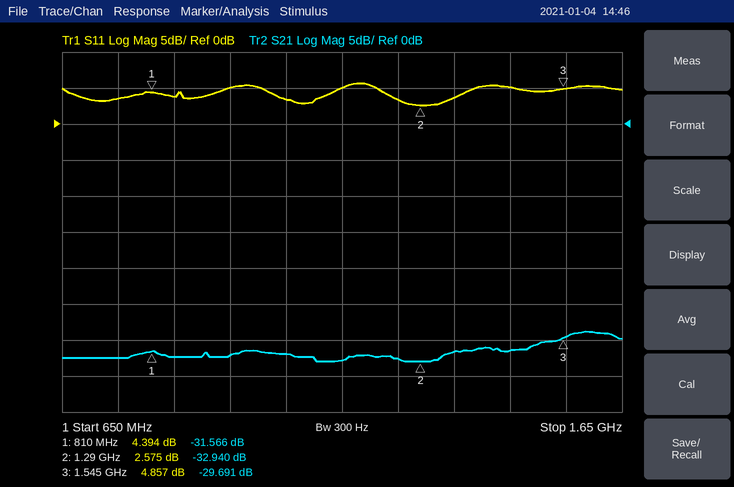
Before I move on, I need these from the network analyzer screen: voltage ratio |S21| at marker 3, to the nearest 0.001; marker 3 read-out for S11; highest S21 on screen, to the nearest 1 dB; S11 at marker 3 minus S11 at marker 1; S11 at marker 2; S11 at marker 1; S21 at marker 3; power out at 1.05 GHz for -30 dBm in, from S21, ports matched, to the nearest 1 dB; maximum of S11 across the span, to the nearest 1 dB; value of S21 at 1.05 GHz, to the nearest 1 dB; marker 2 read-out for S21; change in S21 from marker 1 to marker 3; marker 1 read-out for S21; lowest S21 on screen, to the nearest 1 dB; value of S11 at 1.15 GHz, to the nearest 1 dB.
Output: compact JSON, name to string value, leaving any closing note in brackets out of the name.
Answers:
{"voltage ratio |S21| at marker 3, to the nearest 0.001": "0.033", "marker 3 read-out for S11": "4.857 dB", "highest S21 on screen, to the nearest 1 dB": "-29 dB", "S11 at marker 3 minus S11 at marker 1": "0.463 dB", "S11 at marker 2": "2.575 dB", "S11 at marker 1": "4.394 dB", "S21 at marker 3": "-29.691 dB", "power out at 1.05 GHz for -30 dBm in, from S21, ports matched, to the nearest 1 dB": "-62 dBm", "maximum of S11 across the span, to the nearest 1 dB": "6 dB", "value of S21 at 1.05 GHz, to the nearest 1 dB": "-32 dB", "marker 2 read-out for S21": "-32.940 dB", "change in S21 from marker 1 to marker 3": "1.875 dB", "marker 1 read-out for S21": "-31.566 dB", "lowest S21 on screen, to the nearest 1 dB": "-33 dB", "value of S11 at 1.15 GHz, to the nearest 1 dB": "5 dB"}
